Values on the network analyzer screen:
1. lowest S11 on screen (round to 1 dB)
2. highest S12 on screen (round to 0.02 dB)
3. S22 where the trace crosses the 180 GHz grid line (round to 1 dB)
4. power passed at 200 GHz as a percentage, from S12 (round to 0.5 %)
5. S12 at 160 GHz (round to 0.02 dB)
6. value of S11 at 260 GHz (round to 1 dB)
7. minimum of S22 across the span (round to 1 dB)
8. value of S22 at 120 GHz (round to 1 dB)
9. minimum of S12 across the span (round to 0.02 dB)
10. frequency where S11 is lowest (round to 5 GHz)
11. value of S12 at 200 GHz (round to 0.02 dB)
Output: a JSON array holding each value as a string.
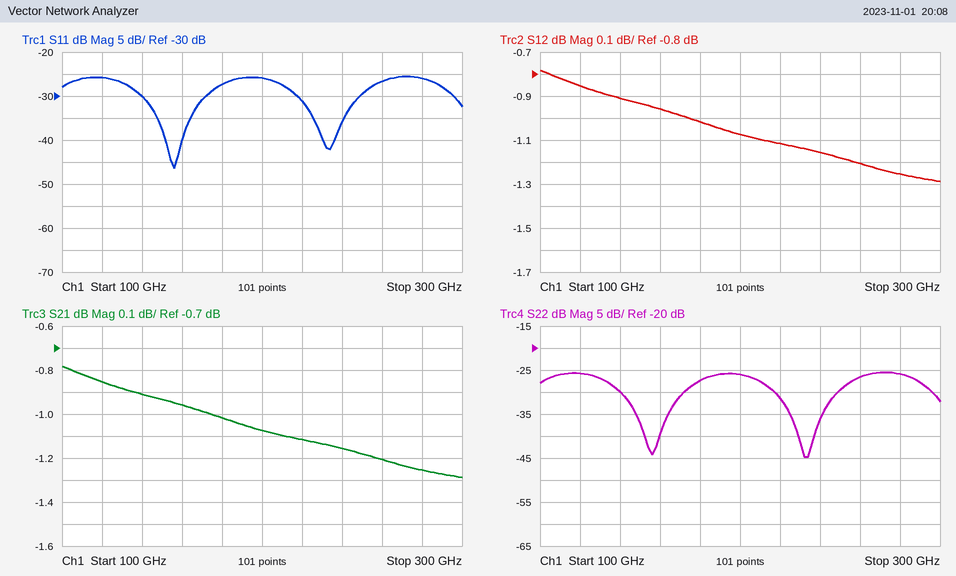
["-46 dB", "-0.78 dB", "-27 dB", "78.0 %", "-0.96 dB", "-27 dB", "-45 dB", "-26 dB", "-1.28 dB", "155 GHz", "-1.08 dB"]
